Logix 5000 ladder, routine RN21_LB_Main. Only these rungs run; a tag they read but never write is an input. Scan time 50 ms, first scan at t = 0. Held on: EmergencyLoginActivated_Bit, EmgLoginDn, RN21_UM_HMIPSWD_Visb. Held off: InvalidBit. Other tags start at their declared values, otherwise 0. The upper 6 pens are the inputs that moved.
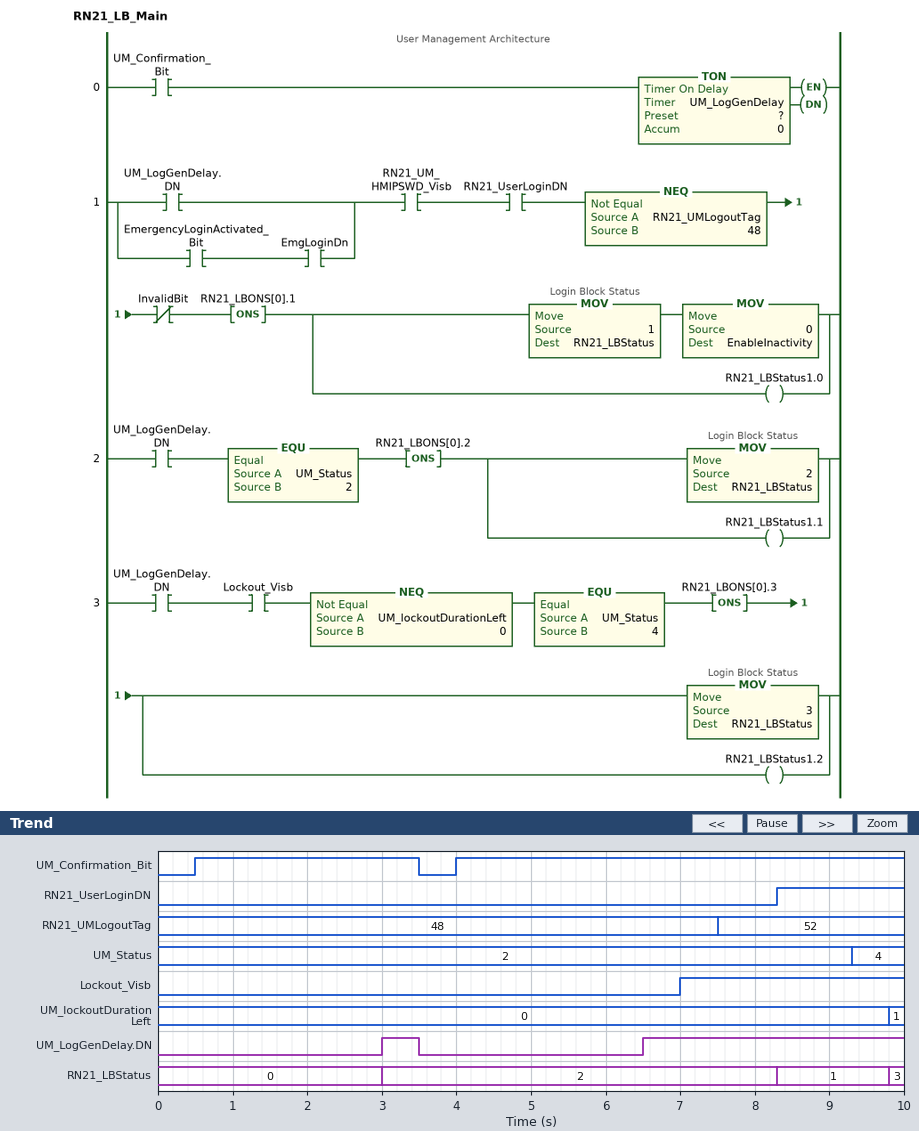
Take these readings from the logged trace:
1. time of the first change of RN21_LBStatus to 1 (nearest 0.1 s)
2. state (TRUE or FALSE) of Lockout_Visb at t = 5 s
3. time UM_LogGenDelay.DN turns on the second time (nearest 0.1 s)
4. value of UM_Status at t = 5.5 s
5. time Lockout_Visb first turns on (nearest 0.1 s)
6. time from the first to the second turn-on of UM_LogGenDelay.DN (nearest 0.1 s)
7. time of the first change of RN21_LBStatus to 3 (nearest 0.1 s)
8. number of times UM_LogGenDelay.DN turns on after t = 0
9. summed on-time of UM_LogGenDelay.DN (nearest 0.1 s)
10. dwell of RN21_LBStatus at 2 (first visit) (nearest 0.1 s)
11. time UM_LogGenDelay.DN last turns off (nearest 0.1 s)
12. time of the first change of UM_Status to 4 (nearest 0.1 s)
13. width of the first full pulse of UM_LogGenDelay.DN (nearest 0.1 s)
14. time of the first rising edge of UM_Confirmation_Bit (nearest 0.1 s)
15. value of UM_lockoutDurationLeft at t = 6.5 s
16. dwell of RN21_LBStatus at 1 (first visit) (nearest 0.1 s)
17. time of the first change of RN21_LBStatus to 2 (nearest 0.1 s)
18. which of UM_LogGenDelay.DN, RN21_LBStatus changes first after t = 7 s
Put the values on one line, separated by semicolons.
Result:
8.3 s; FALSE; 6.5 s; 2; 7.0 s; 3.5 s; 9.8 s; 2; 4.0 s; 5.3 s; 3.5 s; 9.3 s; 0.5 s; 0.5 s; 0; 1.5 s; 3.0 s; RN21_LBStatus
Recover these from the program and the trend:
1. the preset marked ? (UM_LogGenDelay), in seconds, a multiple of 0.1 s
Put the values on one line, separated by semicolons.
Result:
2.5 s
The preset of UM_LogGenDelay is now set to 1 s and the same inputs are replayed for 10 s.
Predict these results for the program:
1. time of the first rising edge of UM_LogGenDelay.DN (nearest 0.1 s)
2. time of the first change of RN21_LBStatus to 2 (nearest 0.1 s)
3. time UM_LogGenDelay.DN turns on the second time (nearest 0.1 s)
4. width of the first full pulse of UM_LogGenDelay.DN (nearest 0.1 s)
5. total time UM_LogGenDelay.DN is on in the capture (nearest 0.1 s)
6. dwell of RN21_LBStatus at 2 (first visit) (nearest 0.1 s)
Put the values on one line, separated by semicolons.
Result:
1.5 s; 1.5 s; 5.0 s; 2.0 s; 7.0 s; 6.8 s
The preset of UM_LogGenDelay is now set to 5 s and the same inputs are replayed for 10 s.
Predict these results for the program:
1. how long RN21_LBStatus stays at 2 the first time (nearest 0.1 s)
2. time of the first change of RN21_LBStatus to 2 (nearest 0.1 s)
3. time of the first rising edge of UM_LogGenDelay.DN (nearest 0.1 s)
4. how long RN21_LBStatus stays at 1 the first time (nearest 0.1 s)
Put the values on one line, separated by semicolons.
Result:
0.8 s; 9.0 s; 9.0 s; 0.7 s
